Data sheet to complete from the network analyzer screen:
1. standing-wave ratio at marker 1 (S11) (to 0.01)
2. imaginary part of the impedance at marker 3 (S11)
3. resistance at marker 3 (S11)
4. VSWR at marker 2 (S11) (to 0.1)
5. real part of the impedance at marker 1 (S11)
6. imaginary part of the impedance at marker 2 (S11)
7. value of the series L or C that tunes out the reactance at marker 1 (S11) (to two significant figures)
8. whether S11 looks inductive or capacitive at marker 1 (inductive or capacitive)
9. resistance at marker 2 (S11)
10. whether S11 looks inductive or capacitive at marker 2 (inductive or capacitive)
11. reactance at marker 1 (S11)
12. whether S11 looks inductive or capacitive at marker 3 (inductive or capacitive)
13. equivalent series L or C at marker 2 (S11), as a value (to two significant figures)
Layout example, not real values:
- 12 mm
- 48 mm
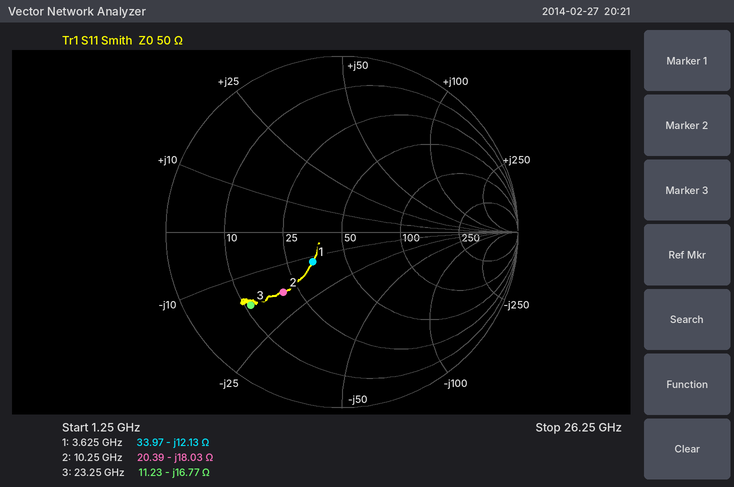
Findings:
- 1.62
- -16.77 Ω
- 11.23 Ω
- 2.8
- 33.97 Ω
- -18.03 Ω
- 530 pH
- capacitive
- 20.39 Ω
- capacitive
- -12.13 Ω
- capacitive
- 860 fF
